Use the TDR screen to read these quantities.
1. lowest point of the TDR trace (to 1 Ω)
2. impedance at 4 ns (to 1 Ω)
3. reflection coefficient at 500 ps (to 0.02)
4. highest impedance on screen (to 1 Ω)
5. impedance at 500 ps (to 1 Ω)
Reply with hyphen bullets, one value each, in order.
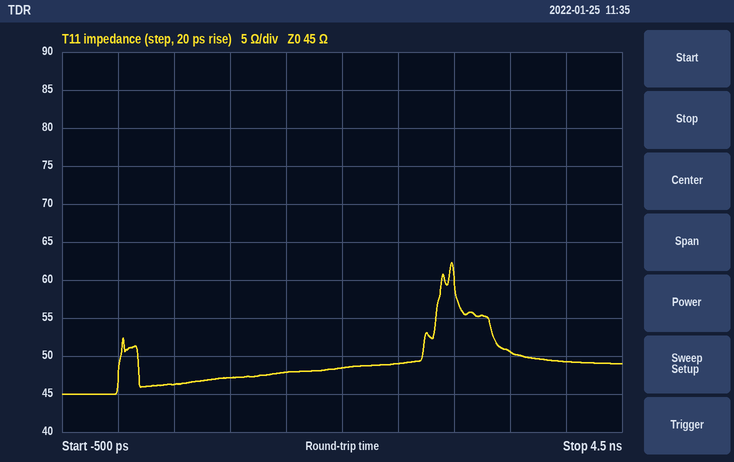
- 45 Ω
- 49 Ω
- +0.02
- 62 Ω
- 46 Ω
